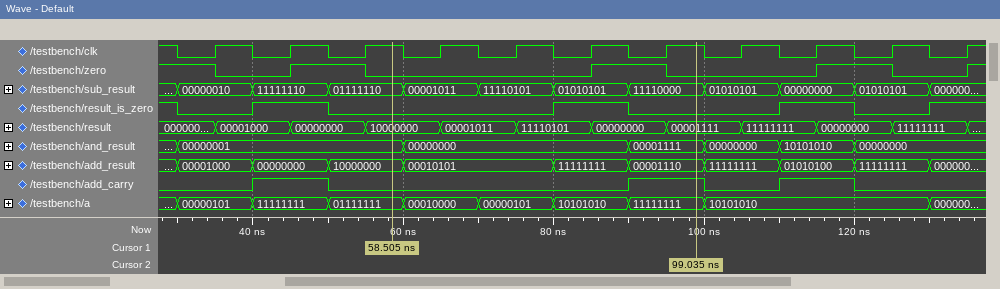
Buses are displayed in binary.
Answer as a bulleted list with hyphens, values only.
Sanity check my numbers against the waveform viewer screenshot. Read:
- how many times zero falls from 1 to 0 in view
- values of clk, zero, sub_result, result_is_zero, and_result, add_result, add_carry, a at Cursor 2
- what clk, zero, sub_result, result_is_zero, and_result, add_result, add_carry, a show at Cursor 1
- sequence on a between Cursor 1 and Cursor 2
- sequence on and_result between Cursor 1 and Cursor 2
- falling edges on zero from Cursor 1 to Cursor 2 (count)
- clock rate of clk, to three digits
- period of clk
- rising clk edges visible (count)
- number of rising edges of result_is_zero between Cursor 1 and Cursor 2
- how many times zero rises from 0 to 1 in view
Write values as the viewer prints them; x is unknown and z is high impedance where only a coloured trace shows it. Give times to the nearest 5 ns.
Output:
- 4
- clk=1, zero=0, sub_result=11110000, result_is_zero=0, and_result=00001111, add_result=00001110, add_carry=1, a=11111111
- clk=1, zero=0, sub_result=01111110, result_is_zero=0, and_result=00000001, add_result=10000000, add_carry=0, a=01111111
- 01111111, 00010000, 00000101, 10101010, 11111111
- 00000001, 00000000, 00001111
- 1
- 100 MHz
- 10 ns
- 11
- 1
- 4
